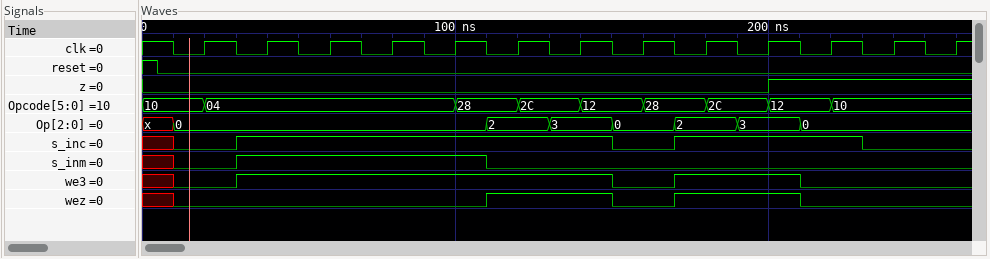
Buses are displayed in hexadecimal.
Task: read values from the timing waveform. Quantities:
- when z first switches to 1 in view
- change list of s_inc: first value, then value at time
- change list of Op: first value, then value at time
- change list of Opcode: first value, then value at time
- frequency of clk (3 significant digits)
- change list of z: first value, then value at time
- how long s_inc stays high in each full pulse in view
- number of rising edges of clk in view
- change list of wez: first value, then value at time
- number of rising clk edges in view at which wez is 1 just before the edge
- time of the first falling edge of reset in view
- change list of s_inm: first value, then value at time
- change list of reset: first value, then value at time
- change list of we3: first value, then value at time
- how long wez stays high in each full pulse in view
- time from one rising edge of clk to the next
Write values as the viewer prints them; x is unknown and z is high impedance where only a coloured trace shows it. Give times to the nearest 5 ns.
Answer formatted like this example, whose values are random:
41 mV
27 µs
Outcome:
200 ns
x, 0 at 10 ns, 1 at 30 ns, 0 at 150 ns, 1 at 170 ns, 0 at 230 ns
x, 0 at 10 ns, 2 at 110 ns, 3 at 130 ns, 0 at 150 ns, 2 at 170 ns, 3 at 190 ns, 0 at 210 ns
10, 04 at 20 ns, 28 at 100 ns, 2C at 120 ns, 12 at 140 ns, 28 at 160 ns, 2C at 180 ns, 12 at 200 ns, 10 at 220 ns
50.0 MHz
0, 1 at 200 ns
120 ns, 60 ns
13
x, 0 at 10 ns, 1 at 110 ns, 0 at 150 ns, 1 at 170 ns, 0 at 210 ns
4
5 ns
x, 0 at 10 ns, 1 at 30 ns, 0 at 110 ns
1, 0 at 5 ns
x, 0 at 10 ns, 1 at 30 ns, 0 at 150 ns, 1 at 170 ns, 0 at 210 ns
40 ns, 40 ns
20 ns
